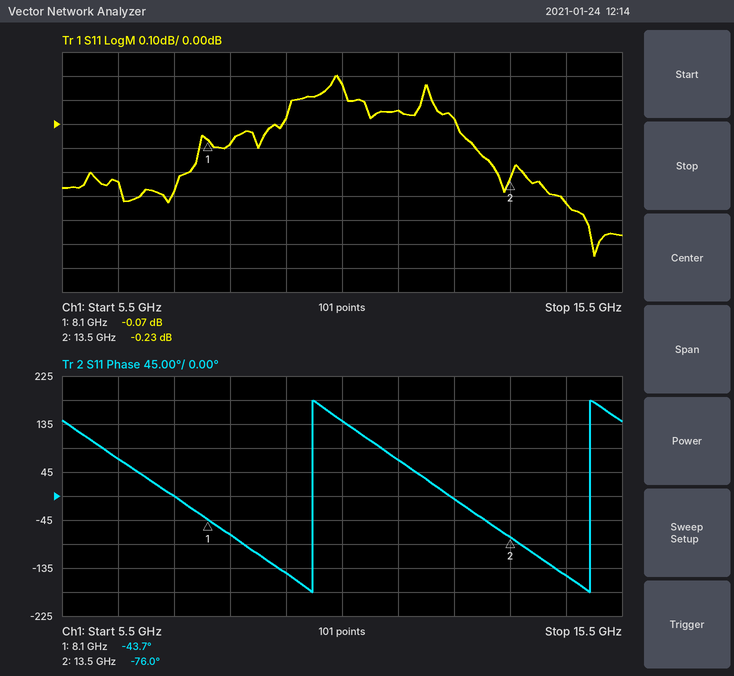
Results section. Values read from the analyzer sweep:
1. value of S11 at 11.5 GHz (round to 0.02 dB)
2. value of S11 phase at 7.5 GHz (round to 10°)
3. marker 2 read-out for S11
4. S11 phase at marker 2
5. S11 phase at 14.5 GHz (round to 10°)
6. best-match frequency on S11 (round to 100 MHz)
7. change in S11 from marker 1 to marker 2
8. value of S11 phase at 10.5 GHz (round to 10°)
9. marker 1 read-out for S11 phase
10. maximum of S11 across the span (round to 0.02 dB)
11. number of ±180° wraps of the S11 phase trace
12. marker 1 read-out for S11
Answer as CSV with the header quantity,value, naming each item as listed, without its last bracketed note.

quantity,value
value of S11 at 11.5 GHz,0.06 dB
value of S11 phase at 7.5 GHz,0°
marker 2 read-out for S11,-0.23 dB
S11 phase at marker 2,-76.0°
S11 phase at 14.5 GHz,-150°
best-match frequency on S11,15.0 GHz
change in S11 from marker 1 to marker 2,-0.16 dB
value of S11 phase at 10.5 GHz,140°
marker 1 read-out for S11 phase,-43.7°
maximum of S11 across the span,0.20 dB
number of ±180° wraps of the S11 phase trace,2
marker 1 read-out for S11,-0.07 dB
